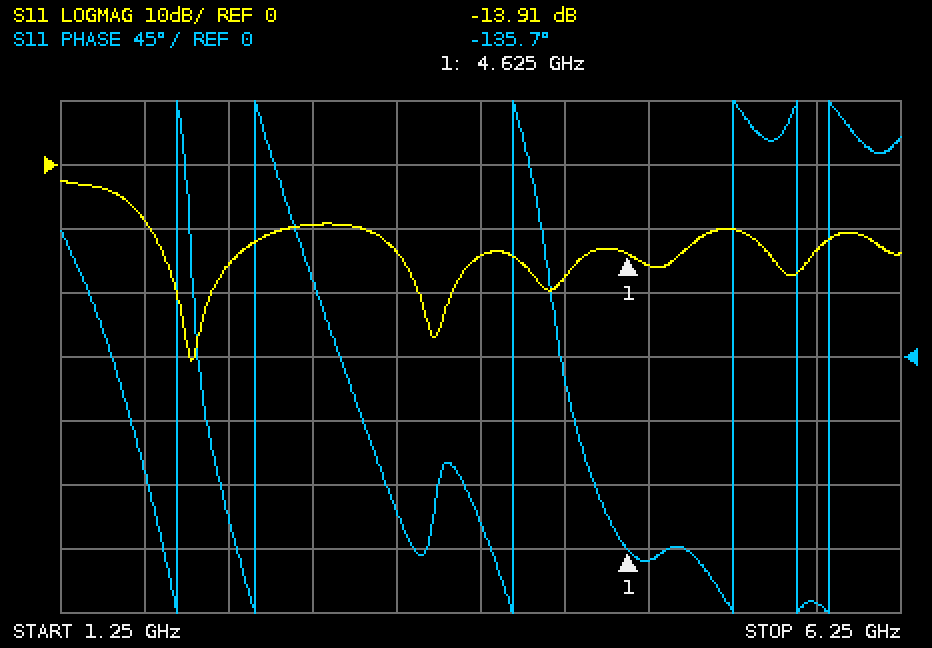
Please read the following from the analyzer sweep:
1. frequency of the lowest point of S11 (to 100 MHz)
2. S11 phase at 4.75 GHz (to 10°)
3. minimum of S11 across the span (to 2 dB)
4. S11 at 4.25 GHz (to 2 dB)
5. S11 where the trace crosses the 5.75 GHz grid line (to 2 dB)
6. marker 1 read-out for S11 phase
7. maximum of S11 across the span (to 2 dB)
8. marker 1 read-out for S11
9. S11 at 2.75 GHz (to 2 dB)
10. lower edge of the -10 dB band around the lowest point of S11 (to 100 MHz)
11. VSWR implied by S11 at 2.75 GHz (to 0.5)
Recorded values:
2.0 GHz
-140°
-30 dB
-18 dB
-14 dB
-135.7°
-2 dB
-13.91 dB
-10 dB
1.8 GHz
2.0
